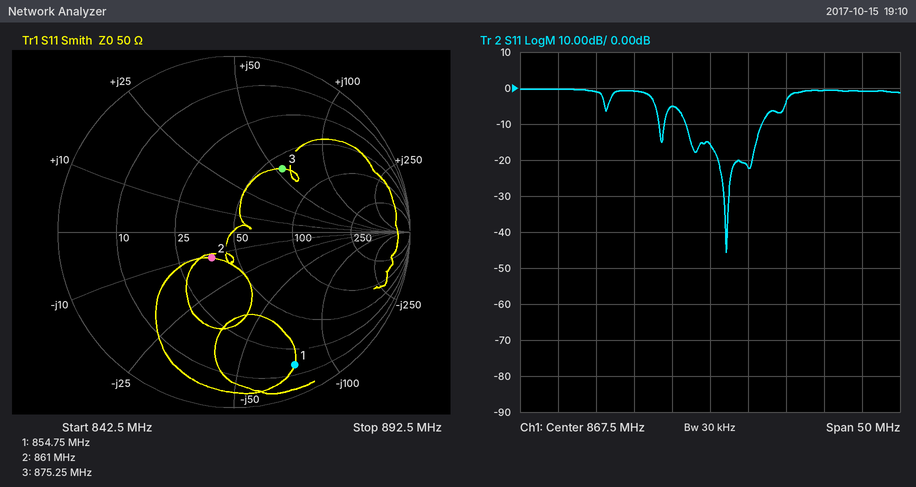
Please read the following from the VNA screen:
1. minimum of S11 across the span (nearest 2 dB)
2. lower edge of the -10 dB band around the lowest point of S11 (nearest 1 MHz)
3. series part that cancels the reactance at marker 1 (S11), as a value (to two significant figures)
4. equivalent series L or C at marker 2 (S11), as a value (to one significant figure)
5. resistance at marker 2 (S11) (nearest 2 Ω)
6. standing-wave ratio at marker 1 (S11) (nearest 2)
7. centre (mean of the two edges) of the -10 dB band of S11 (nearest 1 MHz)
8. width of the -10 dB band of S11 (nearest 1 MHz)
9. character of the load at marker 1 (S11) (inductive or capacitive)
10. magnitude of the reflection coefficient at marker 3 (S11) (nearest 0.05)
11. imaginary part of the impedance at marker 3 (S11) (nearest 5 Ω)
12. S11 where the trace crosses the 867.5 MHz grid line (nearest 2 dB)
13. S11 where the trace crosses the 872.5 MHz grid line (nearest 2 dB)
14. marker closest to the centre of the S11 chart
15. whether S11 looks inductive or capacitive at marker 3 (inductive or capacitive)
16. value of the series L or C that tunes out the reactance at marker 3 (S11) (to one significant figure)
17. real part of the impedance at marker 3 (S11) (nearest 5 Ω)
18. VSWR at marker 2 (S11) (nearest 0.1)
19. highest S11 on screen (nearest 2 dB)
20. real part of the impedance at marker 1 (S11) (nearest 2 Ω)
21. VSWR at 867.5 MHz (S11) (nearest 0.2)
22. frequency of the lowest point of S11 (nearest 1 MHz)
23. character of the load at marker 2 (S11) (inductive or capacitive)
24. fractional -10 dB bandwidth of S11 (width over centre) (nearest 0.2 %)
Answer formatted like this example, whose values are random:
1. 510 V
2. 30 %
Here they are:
1. -46 dB
2. 864 MHz
3. 14 nH
4. 20 pF
5. 38 Ω
6. 10
7. 869 MHz
8. 10 MHz
9. capacitive
10. 0.45
11. +55 Ω
12. -16 dB
13. -22 dB
14. marker 2
15. inductive
16. 3 pF
17. 60 Ω
18. 1.5
19. 0 dB
20. 16 Ω
21. 1.4
22. 870 MHz
23. capacitive
24. 1.2 %
